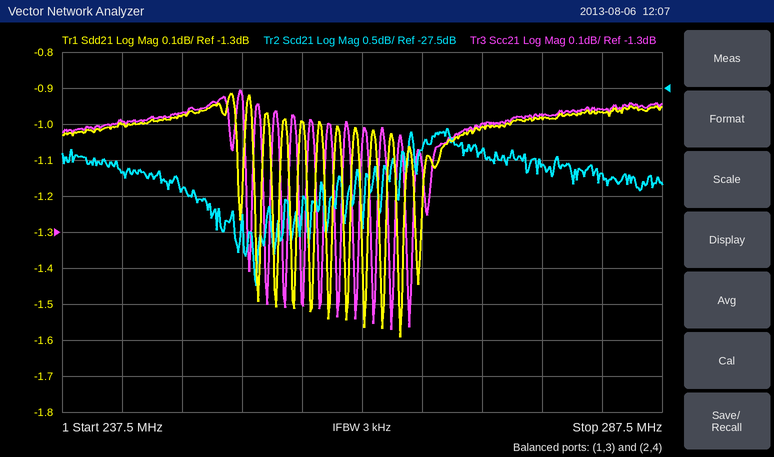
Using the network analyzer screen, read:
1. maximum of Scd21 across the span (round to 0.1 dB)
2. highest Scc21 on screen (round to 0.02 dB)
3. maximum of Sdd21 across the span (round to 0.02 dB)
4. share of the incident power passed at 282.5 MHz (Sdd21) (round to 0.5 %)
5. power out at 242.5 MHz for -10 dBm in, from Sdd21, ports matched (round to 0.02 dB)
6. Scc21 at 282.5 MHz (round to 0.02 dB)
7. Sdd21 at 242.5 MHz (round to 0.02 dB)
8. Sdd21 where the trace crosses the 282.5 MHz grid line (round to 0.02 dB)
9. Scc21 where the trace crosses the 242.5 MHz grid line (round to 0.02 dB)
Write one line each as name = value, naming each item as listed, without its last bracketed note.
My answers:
maximum of Scd21 across the span = -28.1 dB
highest Scc21 on screen = -0.90 dB
maximum of Sdd21 across the span = -0.92 dB
share of the incident power passed at 282.5 MHz (Sdd21) = 80.0 %
power out at 242.5 MHz for -10 dBm in, from Sdd21, ports matched = -11.00 dBm
Scc21 at 282.5 MHz = -0.96 dB
Sdd21 at 242.5 MHz = -1.00 dB
Sdd21 where the trace crosses the 282.5 MHz grid line = -0.96 dB
Scc21 where the trace crosses the 242.5 MHz grid line = -1.00 dB
